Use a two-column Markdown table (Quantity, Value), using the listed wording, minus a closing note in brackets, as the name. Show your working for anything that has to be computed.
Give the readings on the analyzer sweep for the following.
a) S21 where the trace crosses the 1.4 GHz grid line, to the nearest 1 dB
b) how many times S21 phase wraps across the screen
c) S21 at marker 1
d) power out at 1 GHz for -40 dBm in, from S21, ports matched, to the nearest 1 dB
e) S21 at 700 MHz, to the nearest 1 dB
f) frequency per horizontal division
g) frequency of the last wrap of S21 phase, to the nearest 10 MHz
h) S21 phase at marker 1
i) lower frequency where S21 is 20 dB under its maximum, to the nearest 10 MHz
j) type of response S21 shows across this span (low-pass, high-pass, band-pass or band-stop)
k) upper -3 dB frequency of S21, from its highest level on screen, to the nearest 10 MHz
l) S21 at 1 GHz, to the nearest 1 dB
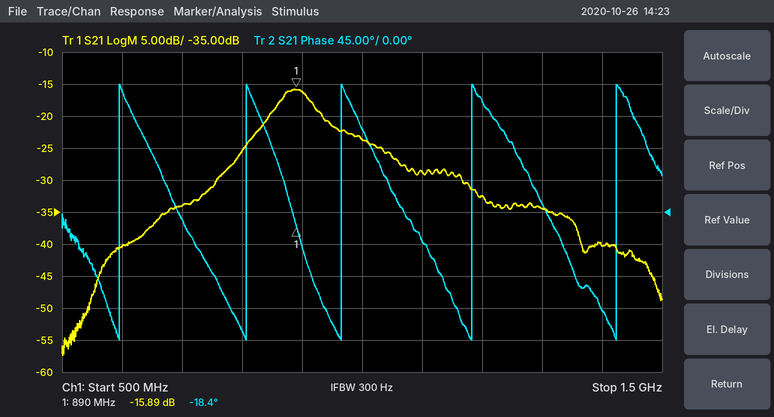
| Quantity | Value |
|---|---|
| S21 where the trace crosses the 1.4 GHz grid line, to the nearest 1 dB | -40 dB |
| how many times S21 phase wraps across the screen | 5 |
| S21 at marker 1 | -15.89 dB |
| power out at 1 GHz for -40 dBm in, from S21, ports matched, to the nearest 1 dB | -40 dBm + (-24 dB) = -64 dBm |
| S21 at 700 MHz, to the nearest 1 dB | -34 dB |
| frequency per horizontal division | 100 MHz |
| frequency of the last wrap of S21 phase, to the nearest 10 MHz | 1.42 GHz |
| S21 phase at marker 1 | -18.4° |
| lower frequency where S21 is 20 dB under its maximum, to the nearest 10 MHz | 660 MHz |
| type of response S21 shows across this span | band-pass |
| upper -3 dB frequency of S21, from its highest level on screen, to the nearest 10 MHz | 920 MHz |
| S21 at 1 GHz, to the nearest 1 dB | -24 dB |
